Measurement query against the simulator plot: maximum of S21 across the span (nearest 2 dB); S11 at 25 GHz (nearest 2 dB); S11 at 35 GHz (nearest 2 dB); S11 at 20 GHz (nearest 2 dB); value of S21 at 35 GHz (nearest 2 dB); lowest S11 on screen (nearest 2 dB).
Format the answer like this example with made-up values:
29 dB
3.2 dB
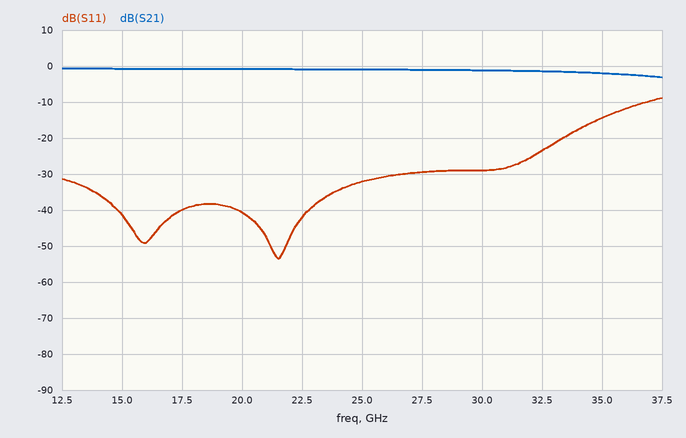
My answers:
0 dB
-32 dB
-14 dB
-40 dB
-2 dB
-54 dB
